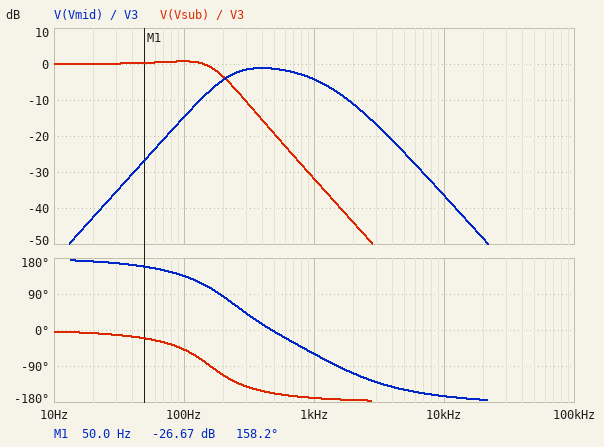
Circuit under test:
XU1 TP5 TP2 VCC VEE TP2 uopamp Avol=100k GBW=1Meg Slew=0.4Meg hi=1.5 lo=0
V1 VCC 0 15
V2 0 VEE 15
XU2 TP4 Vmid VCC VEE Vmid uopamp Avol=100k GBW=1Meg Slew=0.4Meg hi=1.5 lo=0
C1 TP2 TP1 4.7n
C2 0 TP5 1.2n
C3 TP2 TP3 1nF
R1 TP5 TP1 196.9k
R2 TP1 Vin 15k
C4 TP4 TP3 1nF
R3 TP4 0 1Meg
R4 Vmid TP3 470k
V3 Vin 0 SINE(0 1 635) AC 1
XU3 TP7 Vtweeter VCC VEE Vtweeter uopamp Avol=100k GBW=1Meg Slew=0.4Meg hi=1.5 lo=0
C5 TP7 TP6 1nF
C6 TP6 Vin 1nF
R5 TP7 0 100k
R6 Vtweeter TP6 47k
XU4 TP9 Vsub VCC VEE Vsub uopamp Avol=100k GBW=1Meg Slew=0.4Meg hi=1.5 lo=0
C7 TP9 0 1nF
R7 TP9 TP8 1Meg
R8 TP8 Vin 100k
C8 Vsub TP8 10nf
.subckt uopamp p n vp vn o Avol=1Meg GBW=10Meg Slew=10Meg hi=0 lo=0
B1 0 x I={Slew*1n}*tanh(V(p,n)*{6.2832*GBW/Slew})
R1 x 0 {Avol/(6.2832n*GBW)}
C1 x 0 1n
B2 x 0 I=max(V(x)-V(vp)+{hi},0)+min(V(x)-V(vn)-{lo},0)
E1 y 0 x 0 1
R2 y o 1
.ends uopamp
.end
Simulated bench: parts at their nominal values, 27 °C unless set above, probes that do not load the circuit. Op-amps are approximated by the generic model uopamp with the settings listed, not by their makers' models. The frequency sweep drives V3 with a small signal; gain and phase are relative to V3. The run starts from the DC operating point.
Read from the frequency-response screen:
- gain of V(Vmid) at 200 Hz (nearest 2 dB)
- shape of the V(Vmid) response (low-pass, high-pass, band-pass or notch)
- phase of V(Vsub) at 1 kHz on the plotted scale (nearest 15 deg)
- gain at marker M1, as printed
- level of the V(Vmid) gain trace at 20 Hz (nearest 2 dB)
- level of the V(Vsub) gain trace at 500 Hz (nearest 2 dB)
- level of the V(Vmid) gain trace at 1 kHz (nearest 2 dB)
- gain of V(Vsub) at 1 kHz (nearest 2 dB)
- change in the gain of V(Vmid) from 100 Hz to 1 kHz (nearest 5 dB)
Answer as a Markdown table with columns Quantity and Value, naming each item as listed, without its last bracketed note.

| Quantity | Value |
|---|---|
| gain of V(Vmid) at 200 Hz | -4 dB |
| shape of the V(Vmid) response | band-pass |
| phase of V(Vsub) at 1 kHz on the plotted scale | -165 deg |
| gain at marker M1, as printed | -26.67 dB |
| level of the V(Vmid) gain trace at 20 Hz | -42 dB |
| level of the V(Vsub) gain trace at 500 Hz | -20 dB |
| level of the V(Vmid) gain trace at 1 kHz | -4 dB |
| gain of V(Vsub) at 1 kHz | -32 dB |
| change in the gain of V(Vmid) from 100 Hz to 1 kHz | 10 dB |
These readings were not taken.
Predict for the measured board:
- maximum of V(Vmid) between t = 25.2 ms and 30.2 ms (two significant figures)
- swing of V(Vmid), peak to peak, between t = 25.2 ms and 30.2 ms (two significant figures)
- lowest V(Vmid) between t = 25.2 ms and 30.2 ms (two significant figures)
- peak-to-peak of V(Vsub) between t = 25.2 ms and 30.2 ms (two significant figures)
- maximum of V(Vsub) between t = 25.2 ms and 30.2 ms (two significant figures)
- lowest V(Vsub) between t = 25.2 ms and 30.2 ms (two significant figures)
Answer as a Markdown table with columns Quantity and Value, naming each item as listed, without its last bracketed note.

| Quantity | Value |
|---|---|
| maximum of V(Vmid) between t = 25.2 ms and 30.2 ms | 800 mV |
| swing of V(Vmid), peak to peak, between t = 25.2 ms and 30.2 ms | 1.6 V |
| lowest V(Vmid) between t = 25.2 ms and 30.2 ms | -800 mV |
| peak-to-peak of V(Vsub) between t = 25.2 ms and 30.2 ms | 130 mV |
| maximum of V(Vsub) between t = 25.2 ms and 30.2 ms | 64 mV |
| lowest V(Vsub) between t = 25.2 ms and 30.2 ms | -64 mV |
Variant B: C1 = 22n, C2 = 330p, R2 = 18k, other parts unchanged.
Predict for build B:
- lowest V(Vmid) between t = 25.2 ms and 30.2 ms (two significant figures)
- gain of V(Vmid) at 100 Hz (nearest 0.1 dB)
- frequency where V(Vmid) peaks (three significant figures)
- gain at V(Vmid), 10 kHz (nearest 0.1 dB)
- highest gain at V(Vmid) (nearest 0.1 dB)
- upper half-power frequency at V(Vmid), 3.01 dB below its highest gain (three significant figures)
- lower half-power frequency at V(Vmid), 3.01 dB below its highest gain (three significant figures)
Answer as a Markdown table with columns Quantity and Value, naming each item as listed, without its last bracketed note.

| Quantity | Value |
|---|---|
| lowest V(Vmid) between t = 25.2 ms and 30.2 ms | -1.5 V |
| gain of V(Vmid) at 100 Hz | -14.6 dB |
| frequency where V(Vmid) peaks | 941 Hz |
| gain at V(Vmid), 10 kHz | -40.1 dB |
| highest gain at V(Vmid) | 7.3 dB |
| upper half-power frequency at V(Vmid), 3.01 dB below its highest gain | 1.14 kHz |
| lower half-power frequency at V(Vmid), 3.01 dB below its highest gain | 682 Hz |
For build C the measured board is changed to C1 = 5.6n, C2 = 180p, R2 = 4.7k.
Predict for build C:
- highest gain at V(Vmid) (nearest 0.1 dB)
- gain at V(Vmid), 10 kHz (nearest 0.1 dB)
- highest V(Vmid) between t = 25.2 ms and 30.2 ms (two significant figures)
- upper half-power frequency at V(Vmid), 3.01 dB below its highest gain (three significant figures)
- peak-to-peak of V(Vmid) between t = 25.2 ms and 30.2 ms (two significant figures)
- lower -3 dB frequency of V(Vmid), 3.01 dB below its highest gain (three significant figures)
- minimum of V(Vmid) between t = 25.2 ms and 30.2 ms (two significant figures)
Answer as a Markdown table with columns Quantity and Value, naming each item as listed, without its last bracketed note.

| Quantity | Value |
|---|---|
| highest gain at V(Vmid) | 0.4 dB |
| gain at V(Vmid), 10 kHz | -11.0 dB |
| highest V(Vmid) between t = 25.2 ms and 30.2 ms | 1.0 V |
| upper half-power frequency at V(Vmid), 3.01 dB below its highest gain | 5.82 kHz |
| peak-to-peak of V(Vmid) between t = 25.2 ms and 30.2 ms | 2.0 V |
| lower -3 dB frequency of V(Vmid), 3.01 dB below its highest gain | 236 Hz |
| minimum of V(Vmid) between t = 25.2 ms and 30.2 ms | -1.0 V |
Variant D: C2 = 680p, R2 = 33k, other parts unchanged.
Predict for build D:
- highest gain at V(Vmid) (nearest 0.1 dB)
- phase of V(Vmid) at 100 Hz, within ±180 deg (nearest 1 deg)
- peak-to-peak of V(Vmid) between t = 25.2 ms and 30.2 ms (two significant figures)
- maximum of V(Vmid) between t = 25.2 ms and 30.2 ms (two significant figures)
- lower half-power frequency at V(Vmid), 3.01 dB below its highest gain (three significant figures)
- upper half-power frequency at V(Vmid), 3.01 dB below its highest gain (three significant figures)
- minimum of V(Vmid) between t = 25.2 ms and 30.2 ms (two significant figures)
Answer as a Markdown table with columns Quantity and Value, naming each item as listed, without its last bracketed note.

| Quantity | Value |
|---|---|
| highest gain at V(Vmid) | 0.8 dB |
| phase of V(Vmid) at 100 Hz, within ±180 deg | 138 deg |
| peak-to-peak of V(Vmid) between t = 25.2 ms and 30.2 ms | 2.2 V |
| maximum of V(Vmid) between t = 25.2 ms and 30.2 ms | 1.1 V |
| lower half-power frequency at V(Vmid), 3.01 dB below its highest gain | 243 Hz |
| upper half-power frequency at V(Vmid), 3.01 dB below its highest gain | 1.27 kHz |
| minimum of V(Vmid) between t = 25.2 ms and 30.2 ms | -1.1 V |
